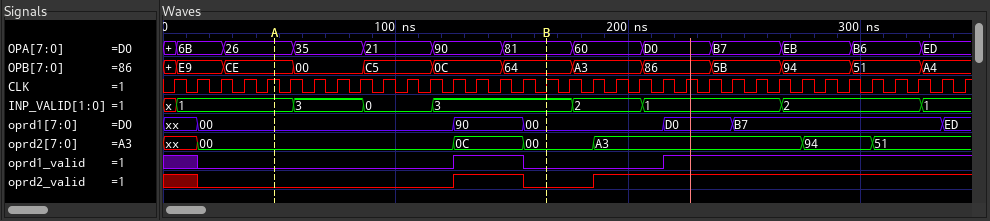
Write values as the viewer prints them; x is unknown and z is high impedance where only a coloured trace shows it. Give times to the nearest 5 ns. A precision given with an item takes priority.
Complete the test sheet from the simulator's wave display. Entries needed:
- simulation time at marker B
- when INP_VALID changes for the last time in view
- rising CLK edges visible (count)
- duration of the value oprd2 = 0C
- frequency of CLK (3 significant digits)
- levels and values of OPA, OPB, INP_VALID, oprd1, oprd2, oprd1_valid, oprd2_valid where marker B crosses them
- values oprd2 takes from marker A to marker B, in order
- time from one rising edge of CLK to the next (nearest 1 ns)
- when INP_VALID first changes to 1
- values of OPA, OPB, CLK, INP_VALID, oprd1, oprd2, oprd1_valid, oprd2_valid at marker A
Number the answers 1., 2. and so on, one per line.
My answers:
1. 165 ns
2. 325 ns
3. 35
4. 30 ns
5. 100 MHz
6. OPA=81, OPB=64, INP_VALID=3, oprd1=00, oprd2=00, oprd1_valid=0, oprd2_valid=0
7. 00, 0C, 00
8. 10 ns
9. 5 ns
10. OPA=26, OPB=CE, CLK=1, INP_VALID=1, oprd1=00, oprd2=00, oprd1_valid=0, oprd2_valid=0
